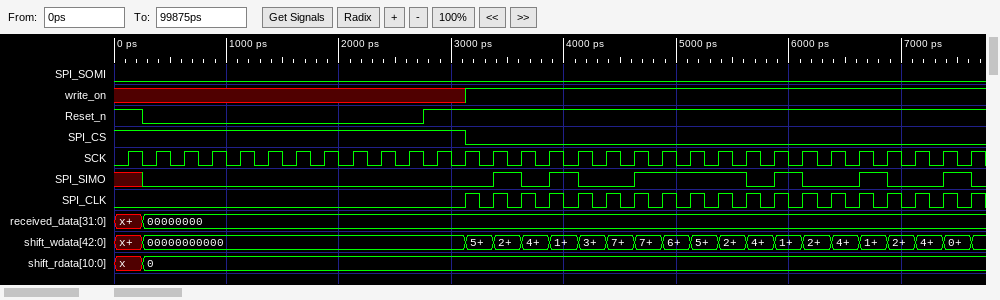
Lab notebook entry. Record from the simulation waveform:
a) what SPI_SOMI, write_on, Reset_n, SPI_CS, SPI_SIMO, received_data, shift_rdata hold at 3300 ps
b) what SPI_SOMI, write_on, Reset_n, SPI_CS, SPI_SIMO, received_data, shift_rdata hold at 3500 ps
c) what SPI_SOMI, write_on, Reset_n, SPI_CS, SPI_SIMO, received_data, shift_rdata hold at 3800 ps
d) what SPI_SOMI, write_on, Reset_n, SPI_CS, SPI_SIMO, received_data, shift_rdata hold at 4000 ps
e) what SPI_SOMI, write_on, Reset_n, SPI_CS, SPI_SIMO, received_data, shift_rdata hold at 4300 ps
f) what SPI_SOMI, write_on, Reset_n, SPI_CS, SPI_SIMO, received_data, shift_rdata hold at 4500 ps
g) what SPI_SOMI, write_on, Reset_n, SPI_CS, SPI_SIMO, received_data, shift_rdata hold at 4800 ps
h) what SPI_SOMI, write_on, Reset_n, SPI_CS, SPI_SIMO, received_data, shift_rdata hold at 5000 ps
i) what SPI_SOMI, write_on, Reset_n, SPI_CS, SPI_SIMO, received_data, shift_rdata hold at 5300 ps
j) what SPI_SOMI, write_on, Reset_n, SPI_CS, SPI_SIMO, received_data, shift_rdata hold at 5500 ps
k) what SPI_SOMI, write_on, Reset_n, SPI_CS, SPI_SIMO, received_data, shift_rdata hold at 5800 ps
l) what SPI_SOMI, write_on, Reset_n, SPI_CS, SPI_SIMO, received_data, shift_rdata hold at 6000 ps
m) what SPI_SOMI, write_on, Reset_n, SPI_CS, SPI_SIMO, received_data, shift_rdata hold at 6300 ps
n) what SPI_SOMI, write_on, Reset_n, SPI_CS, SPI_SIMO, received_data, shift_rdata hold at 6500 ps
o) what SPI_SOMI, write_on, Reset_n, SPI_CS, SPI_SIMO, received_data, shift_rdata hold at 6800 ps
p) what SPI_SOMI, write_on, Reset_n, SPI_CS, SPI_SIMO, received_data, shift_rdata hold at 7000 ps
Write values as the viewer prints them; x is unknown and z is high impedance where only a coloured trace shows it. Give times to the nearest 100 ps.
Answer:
SPI_SOMI=0, write_on=1, Reset_n=1, SPI_CS=0, SPI_SIMO=0, received_data=00000000, shift_rdata=0
SPI_SOMI=0, write_on=1, Reset_n=1, SPI_CS=0, SPI_SIMO=1, received_data=00000000, shift_rdata=0
SPI_SOMI=0, write_on=1, Reset_n=1, SPI_CS=0, SPI_SIMO=0, received_data=00000000, shift_rdata=0
SPI_SOMI=0, write_on=1, Reset_n=1, SPI_CS=0, SPI_SIMO=1, received_data=00000000, shift_rdata=0
SPI_SOMI=0, write_on=1, Reset_n=1, SPI_CS=0, SPI_SIMO=0, received_data=00000000, shift_rdata=0
SPI_SOMI=0, write_on=1, Reset_n=1, SPI_CS=0, SPI_SIMO=0, received_data=00000000, shift_rdata=0
SPI_SOMI=0, write_on=1, Reset_n=1, SPI_CS=0, SPI_SIMO=1, received_data=00000000, shift_rdata=0
SPI_SOMI=0, write_on=1, Reset_n=1, SPI_CS=0, SPI_SIMO=1, received_data=00000000, shift_rdata=0
SPI_SOMI=0, write_on=1, Reset_n=1, SPI_CS=0, SPI_SIMO=1, received_data=00000000, shift_rdata=0
SPI_SOMI=0, write_on=1, Reset_n=1, SPI_CS=0, SPI_SIMO=1, received_data=00000000, shift_rdata=0
SPI_SOMI=0, write_on=1, Reset_n=1, SPI_CS=0, SPI_SIMO=0, received_data=00000000, shift_rdata=0
SPI_SOMI=0, write_on=1, Reset_n=1, SPI_CS=0, SPI_SIMO=1, received_data=00000000, shift_rdata=0
SPI_SOMI=0, write_on=1, Reset_n=1, SPI_CS=0, SPI_SIMO=0, received_data=00000000, shift_rdata=0
SPI_SOMI=0, write_on=1, Reset_n=1, SPI_CS=0, SPI_SIMO=0, received_data=00000000, shift_rdata=0
SPI_SOMI=0, write_on=1, Reset_n=1, SPI_CS=0, SPI_SIMO=1, received_data=00000000, shift_rdata=0
SPI_SOMI=0, write_on=1, Reset_n=1, SPI_CS=0, SPI_SIMO=0, received_data=00000000, shift_rdata=0
